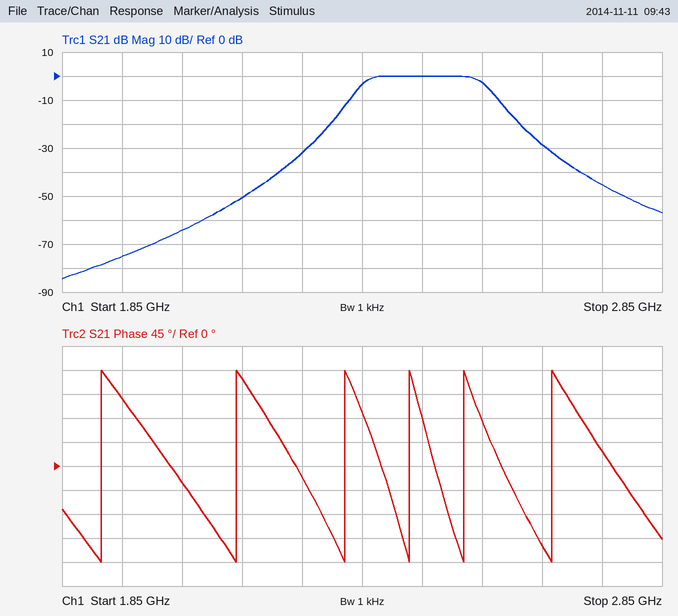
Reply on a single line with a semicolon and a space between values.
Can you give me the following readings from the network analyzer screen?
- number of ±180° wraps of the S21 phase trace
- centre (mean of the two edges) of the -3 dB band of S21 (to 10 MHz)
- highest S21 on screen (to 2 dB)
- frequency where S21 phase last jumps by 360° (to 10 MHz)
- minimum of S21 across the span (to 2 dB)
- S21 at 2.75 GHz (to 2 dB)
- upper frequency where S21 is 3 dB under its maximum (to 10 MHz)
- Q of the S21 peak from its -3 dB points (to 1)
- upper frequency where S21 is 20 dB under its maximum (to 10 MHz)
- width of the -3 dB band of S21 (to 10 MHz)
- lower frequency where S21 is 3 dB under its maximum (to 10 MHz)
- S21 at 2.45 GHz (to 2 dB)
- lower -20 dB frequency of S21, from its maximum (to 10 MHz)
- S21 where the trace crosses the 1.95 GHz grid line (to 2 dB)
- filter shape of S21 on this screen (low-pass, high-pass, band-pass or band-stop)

6; 2.45 GHz; 0 dB; 2.67 GHz; -84 dB; -46 dB; 2.55 GHz; 12; 2.61 GHz; 200 MHz; 2.35 GHz; 0 dB; 2.30 GHz; -76 dB; band-pass
